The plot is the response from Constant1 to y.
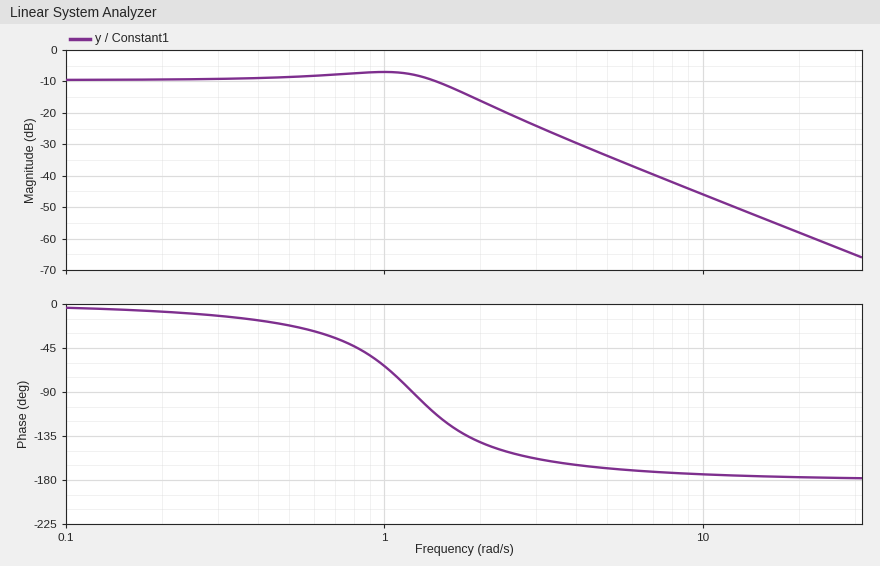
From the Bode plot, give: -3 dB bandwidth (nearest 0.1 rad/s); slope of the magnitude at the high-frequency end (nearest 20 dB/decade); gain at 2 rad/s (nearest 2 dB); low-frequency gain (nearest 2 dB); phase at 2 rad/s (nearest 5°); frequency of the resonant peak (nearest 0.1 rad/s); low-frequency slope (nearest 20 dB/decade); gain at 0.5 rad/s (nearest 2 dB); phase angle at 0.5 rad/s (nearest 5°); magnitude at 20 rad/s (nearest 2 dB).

1.7 rad/s
-40 dB/decade
-16 dB
-10 dB
-140°
1.0 rad/s
0 dB/decade
-8 dB
-20°
-58 dB
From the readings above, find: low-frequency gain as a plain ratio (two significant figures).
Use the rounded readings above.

0.32
